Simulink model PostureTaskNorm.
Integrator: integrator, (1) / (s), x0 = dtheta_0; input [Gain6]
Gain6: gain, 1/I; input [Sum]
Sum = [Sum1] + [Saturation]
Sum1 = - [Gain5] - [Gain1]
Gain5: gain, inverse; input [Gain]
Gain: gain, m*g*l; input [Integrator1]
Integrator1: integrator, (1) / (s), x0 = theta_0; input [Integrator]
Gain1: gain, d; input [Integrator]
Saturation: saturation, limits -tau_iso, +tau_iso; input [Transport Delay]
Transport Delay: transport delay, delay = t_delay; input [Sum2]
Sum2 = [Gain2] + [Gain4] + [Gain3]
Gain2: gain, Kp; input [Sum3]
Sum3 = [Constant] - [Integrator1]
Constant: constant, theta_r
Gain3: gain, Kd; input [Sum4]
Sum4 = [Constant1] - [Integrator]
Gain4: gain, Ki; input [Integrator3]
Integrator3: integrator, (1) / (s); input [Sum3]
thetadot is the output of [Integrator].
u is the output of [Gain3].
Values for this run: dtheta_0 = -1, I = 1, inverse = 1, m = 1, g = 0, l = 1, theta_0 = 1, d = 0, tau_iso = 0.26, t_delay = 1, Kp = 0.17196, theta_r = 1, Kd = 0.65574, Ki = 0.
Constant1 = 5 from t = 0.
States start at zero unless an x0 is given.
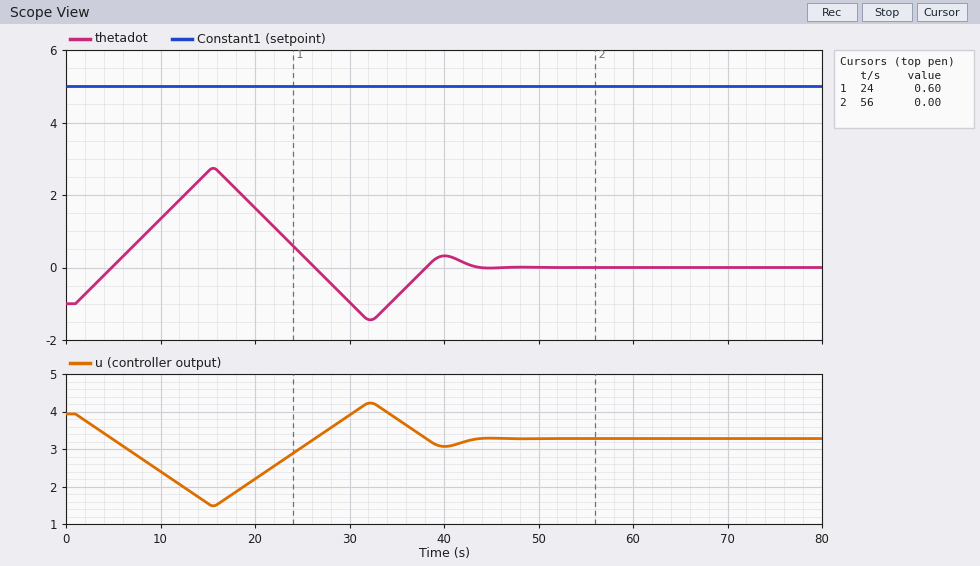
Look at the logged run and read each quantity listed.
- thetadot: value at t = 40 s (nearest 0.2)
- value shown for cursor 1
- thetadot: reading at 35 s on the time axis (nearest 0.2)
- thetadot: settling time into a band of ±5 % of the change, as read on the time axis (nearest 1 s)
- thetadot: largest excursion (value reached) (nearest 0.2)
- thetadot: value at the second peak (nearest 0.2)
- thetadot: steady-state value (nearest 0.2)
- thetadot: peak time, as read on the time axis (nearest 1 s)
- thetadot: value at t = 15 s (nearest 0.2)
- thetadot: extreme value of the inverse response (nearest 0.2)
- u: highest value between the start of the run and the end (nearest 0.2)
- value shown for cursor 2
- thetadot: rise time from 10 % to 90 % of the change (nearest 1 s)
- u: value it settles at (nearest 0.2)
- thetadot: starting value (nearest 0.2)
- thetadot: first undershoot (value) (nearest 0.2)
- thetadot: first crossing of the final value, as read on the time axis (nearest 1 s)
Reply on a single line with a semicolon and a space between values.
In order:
0.4; 0.60; -0.8; 43 s; 2.8; 0.4; 0.0; 16 s; 2.6; -1.4; 4.2; 0.00; 3 s; 3.2; -1.0; -1.4; 5 s
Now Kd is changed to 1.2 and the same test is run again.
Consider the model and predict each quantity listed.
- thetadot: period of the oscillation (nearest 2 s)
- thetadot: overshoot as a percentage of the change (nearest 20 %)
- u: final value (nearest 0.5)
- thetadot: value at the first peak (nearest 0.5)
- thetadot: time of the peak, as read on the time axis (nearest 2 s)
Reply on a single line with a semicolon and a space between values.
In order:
18 s; 320 %; 6.0; 3.0; 18 s
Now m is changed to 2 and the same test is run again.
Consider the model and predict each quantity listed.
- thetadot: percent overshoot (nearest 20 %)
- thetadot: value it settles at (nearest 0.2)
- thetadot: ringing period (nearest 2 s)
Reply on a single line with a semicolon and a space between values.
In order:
280 %; 0.0; 24 s
